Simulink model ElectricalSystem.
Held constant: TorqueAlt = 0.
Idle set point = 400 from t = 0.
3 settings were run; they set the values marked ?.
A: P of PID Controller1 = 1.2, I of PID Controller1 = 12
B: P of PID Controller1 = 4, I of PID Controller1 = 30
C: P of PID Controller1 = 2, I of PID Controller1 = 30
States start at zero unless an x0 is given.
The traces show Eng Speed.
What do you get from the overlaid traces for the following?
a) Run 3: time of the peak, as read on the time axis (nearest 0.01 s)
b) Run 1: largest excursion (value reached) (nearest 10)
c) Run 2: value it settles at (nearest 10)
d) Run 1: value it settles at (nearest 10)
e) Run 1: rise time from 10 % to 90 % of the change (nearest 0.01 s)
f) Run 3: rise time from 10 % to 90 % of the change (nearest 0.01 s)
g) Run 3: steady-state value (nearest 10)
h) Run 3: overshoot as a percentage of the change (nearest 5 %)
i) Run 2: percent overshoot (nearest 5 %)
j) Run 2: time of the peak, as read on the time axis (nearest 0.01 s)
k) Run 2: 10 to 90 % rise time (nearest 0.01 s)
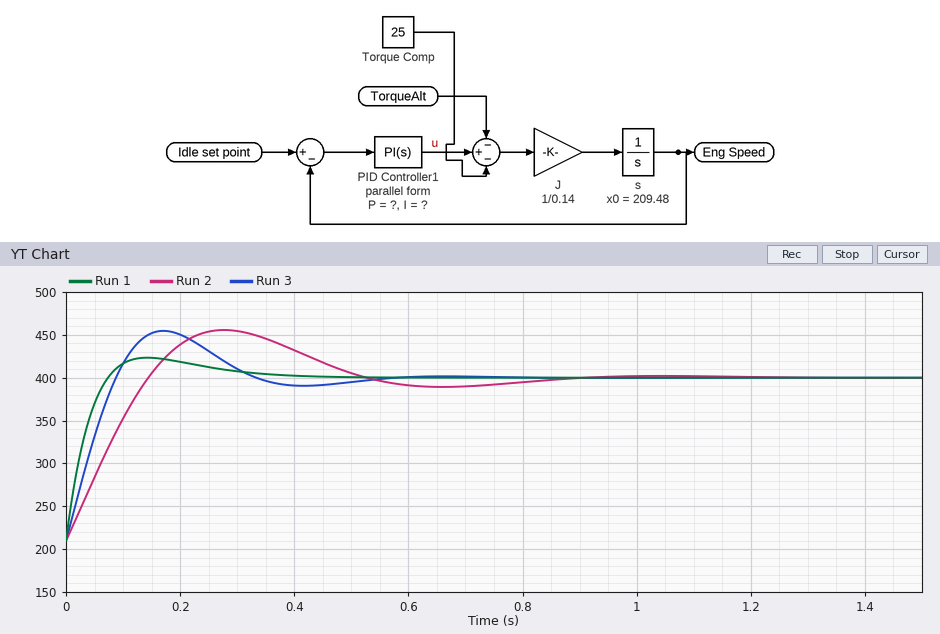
0.17 s
420
400
400
0.05 s
0.07 s
400
30 %
30 %
0.28 s
0.11 s
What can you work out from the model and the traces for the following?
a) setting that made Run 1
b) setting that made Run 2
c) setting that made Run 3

B
A
C
